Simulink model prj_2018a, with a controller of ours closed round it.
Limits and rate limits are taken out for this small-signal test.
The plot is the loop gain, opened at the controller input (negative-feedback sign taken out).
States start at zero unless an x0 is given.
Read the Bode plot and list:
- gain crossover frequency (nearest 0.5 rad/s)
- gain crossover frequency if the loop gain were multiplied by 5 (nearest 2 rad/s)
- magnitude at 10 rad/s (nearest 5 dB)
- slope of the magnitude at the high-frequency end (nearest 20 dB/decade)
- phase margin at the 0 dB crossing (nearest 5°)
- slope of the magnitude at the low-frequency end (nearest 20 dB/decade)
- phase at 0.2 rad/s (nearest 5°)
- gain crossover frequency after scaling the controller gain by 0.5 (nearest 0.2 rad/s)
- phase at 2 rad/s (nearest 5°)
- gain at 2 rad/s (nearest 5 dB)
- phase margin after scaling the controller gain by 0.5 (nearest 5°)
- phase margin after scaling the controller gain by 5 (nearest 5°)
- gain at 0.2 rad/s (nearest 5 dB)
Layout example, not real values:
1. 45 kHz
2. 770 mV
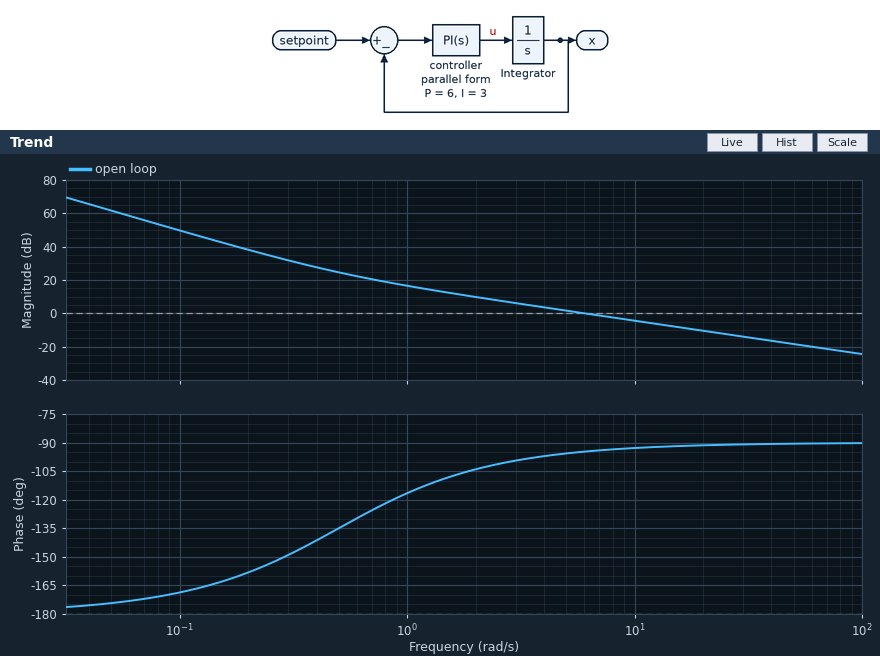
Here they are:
1. 6.0 rad/s
2. 30 rad/s
3. -5 dB
4. -20 dB/decade
5. 85°
6. -40 dB/decade
7. -160°
8. 3.0 rad/s
9. -105°
10. 10 dB
11. 80°
12. 90°
13. 40 dB
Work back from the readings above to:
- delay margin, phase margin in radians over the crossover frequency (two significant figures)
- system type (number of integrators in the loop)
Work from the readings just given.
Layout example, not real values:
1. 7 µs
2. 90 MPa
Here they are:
1. 0.25 s
2. 2
